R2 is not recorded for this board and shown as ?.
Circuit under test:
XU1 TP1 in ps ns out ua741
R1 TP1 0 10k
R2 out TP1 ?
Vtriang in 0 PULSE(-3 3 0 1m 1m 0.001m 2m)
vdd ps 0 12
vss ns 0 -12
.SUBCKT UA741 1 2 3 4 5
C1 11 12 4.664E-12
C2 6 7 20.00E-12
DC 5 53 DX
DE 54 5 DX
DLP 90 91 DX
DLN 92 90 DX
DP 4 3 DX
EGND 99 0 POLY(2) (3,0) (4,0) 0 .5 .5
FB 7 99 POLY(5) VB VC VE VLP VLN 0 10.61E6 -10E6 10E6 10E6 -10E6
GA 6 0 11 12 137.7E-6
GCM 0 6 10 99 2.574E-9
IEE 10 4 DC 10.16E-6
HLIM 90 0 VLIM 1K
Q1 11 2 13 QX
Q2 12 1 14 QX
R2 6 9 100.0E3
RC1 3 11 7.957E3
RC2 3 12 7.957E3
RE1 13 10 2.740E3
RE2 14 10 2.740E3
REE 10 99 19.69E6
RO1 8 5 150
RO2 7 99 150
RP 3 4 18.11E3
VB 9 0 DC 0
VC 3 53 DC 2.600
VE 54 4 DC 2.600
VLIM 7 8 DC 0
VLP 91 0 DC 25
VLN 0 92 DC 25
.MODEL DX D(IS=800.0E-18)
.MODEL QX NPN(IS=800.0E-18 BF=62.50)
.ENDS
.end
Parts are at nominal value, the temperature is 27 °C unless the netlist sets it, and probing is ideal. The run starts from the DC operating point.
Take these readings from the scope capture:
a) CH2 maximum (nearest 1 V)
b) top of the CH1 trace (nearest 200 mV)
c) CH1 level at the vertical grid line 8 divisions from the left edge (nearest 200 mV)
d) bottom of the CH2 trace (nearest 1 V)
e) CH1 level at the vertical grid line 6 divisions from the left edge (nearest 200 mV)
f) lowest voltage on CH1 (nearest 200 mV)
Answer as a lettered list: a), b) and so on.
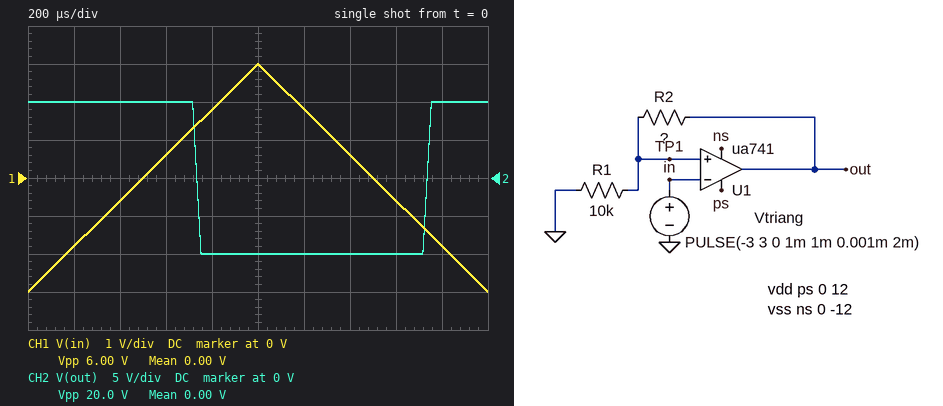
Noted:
a) 10 V
b) 3.0 V
c) -600 mV
d) -10 V
e) 1.8 V
f) -3.0 V
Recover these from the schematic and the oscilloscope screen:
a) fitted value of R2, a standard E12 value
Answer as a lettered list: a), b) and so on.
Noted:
a) 68 kΩ
